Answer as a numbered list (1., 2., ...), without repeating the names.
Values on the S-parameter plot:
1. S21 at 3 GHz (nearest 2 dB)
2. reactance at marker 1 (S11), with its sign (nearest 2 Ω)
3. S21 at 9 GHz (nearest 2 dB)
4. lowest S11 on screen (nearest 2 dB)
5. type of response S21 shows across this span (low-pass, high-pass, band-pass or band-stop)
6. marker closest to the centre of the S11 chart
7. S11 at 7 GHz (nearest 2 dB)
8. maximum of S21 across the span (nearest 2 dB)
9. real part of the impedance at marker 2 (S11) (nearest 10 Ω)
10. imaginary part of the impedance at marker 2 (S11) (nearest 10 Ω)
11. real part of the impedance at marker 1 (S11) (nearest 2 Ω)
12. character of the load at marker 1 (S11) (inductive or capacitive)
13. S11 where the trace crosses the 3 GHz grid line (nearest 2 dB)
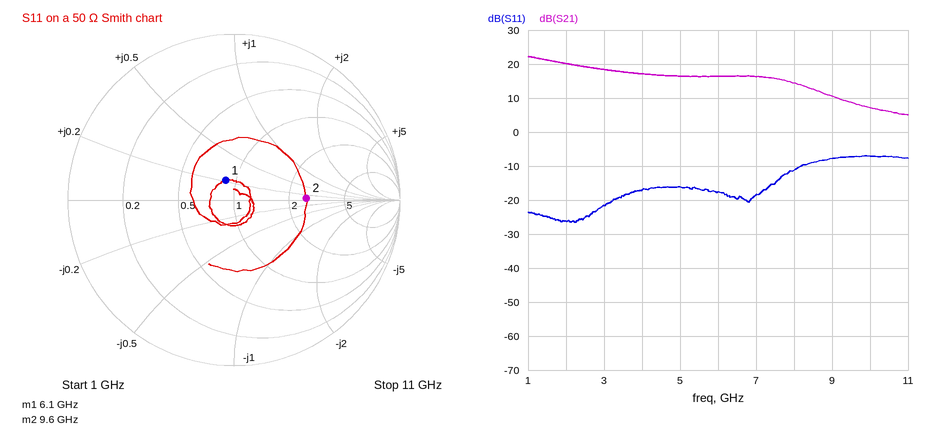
1. 18 dB
2. +10 Ω
3. 10 dB
4. -26 dB
5. low-pass
6. marker 1
7. -18 dB
8. 22 dB
9. 130 Ω
10. 0 Ω
11. 44 Ω
12. inductive
13. -22 dB
